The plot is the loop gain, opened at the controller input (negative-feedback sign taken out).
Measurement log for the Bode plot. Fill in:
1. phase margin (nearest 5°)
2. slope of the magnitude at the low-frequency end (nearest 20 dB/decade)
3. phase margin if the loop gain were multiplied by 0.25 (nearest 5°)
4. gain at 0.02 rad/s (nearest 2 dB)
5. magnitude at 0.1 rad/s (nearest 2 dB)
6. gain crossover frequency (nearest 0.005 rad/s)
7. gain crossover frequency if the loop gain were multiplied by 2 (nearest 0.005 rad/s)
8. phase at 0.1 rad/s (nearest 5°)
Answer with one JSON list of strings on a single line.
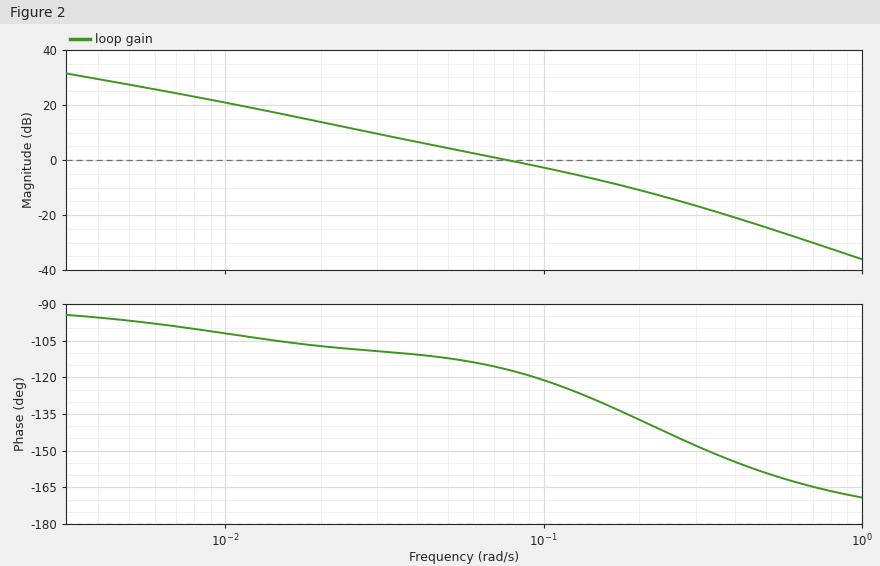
["65°", "-20 dB/decade", "70°", "14 dB", "-2 dB", "0.075 rad/s", "0.135 rad/s", "-120°"]
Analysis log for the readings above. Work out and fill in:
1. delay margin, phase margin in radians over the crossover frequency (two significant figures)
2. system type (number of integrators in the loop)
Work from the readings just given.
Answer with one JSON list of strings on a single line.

["15 s", "1"]
